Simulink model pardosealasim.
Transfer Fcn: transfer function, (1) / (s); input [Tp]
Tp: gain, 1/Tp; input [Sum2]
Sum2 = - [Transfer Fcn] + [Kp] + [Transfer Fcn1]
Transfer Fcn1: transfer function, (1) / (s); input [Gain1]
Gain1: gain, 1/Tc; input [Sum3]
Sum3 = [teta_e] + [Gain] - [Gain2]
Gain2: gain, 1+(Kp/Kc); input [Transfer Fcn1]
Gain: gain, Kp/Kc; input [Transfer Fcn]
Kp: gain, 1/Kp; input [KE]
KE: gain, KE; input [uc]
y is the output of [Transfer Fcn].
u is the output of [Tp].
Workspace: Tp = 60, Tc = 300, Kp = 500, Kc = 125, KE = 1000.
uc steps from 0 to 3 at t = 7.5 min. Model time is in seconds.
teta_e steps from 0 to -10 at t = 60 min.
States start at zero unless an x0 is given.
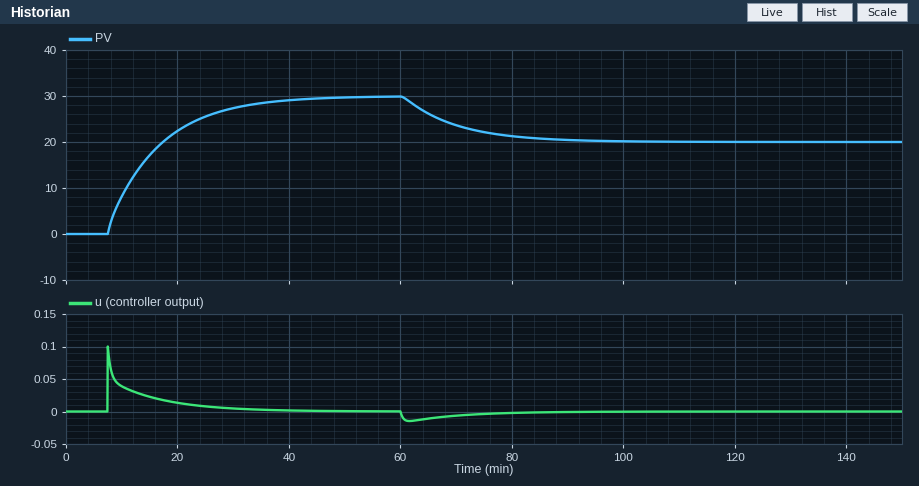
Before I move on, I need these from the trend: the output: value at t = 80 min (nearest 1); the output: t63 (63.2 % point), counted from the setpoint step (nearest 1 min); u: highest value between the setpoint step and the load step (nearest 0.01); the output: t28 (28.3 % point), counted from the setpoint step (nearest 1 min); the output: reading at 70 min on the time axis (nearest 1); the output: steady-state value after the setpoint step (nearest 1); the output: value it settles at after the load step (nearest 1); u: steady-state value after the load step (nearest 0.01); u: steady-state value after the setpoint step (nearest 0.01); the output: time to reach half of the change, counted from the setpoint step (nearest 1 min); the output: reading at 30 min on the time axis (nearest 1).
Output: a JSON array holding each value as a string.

["21", "9 min", "0.10", "3 min", "24", "30", "20", "0.00", "0.00", "6 min", "27"]
